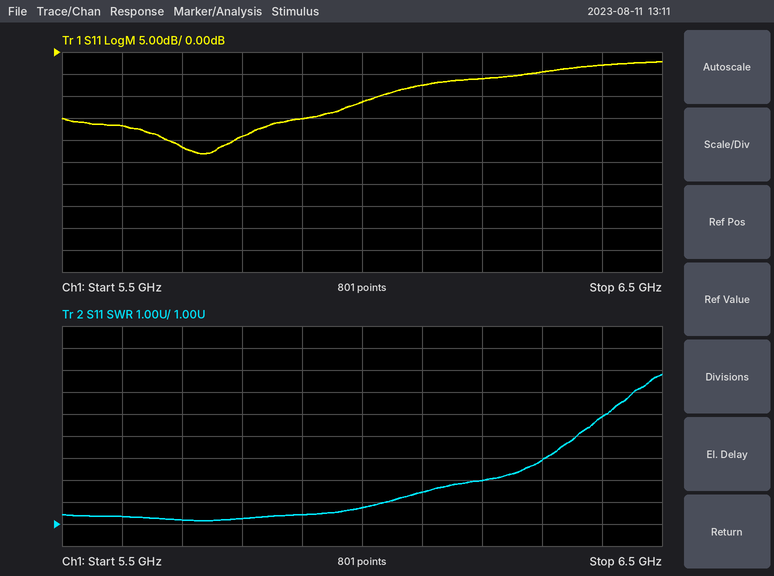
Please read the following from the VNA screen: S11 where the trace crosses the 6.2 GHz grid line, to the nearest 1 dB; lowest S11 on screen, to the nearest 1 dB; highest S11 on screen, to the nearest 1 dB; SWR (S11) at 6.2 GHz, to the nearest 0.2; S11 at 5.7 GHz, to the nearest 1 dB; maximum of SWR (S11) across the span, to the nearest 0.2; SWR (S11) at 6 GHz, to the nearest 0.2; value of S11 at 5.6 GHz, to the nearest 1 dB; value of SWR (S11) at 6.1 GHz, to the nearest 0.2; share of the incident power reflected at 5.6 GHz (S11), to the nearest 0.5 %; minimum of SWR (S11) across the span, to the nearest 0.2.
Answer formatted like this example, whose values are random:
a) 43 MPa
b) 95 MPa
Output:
a) -6 dB
b) -23 dB
c) -2 dB
d) 3.0
e) -22 dB
f) 7.8
g) 1.8
h) -17 dB
i) 2.4
j) 2.0 %
k) 1.2
